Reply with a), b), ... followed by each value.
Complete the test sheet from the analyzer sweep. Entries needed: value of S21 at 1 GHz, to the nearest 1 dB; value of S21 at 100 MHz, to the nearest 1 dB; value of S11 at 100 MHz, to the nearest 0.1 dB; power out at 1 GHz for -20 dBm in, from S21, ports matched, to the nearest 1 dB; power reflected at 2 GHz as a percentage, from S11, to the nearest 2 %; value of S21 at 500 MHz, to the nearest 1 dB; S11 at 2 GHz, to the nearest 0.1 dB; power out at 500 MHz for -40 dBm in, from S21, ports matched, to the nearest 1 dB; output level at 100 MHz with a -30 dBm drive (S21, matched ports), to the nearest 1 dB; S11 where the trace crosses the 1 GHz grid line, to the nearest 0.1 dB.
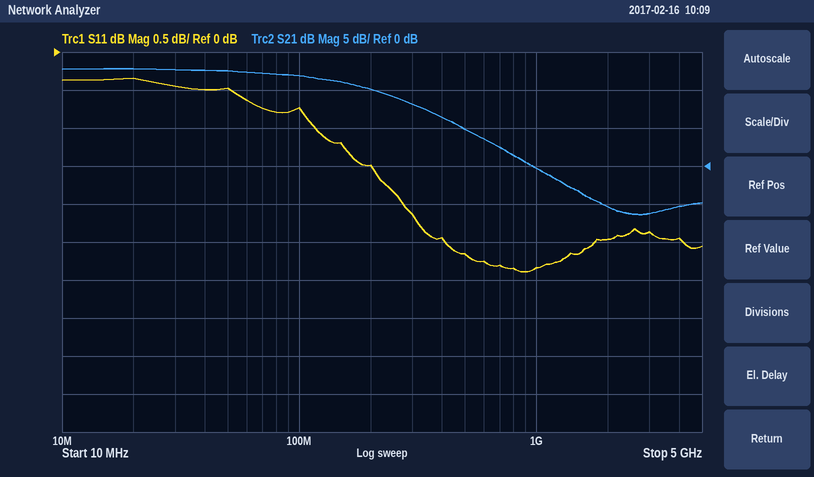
a) 0 dB
b) 12 dB
c) -0.7 dB
d) -20 dBm
e) 56 %
f) 5 dB
g) -2.5 dB
h) -35 dBm
i) -18 dBm
j) -2.8 dB
